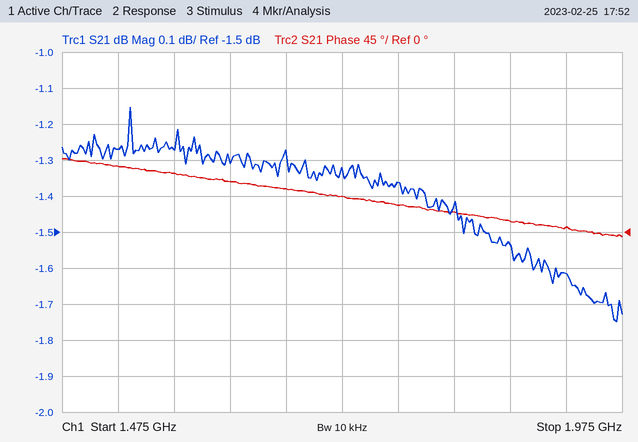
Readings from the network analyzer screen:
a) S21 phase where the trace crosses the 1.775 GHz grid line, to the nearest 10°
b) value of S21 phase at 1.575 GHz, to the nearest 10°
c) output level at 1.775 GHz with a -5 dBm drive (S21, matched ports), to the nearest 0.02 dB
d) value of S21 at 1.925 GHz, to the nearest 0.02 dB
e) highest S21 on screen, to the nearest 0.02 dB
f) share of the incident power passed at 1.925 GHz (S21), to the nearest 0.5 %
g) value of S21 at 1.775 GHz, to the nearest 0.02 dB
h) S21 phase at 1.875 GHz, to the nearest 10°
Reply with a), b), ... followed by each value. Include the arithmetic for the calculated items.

a) 30°
b) 70°
c) -5 dBm + (-1.36 dB) = -6.36 dBm
d) -1.62 dB
e) -1.16 dB
f) 10^(-1.62/10) ≈ 68.9 %, so 69.0 % to the nearest 0.5 %
g) -1.36 dB
h) 10°
